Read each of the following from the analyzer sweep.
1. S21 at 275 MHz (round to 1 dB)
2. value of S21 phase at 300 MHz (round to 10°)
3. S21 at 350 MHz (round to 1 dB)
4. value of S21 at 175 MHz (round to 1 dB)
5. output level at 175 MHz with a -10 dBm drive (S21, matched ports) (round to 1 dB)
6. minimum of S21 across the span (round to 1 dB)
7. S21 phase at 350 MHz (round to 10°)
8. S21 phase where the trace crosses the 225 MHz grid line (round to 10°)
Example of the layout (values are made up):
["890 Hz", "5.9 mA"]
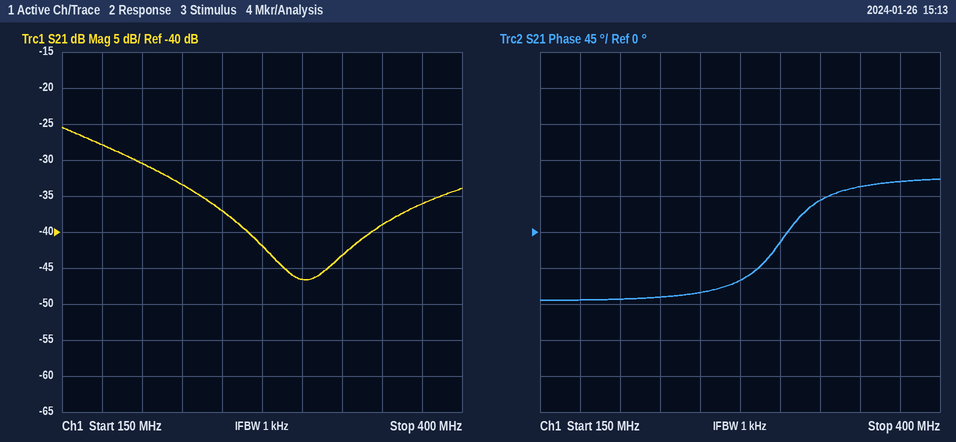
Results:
["-42 dB", "-10°", "-39 dB", "-28 dB", "-38 dBm", "-47 dB", "60°", "-80°"]
